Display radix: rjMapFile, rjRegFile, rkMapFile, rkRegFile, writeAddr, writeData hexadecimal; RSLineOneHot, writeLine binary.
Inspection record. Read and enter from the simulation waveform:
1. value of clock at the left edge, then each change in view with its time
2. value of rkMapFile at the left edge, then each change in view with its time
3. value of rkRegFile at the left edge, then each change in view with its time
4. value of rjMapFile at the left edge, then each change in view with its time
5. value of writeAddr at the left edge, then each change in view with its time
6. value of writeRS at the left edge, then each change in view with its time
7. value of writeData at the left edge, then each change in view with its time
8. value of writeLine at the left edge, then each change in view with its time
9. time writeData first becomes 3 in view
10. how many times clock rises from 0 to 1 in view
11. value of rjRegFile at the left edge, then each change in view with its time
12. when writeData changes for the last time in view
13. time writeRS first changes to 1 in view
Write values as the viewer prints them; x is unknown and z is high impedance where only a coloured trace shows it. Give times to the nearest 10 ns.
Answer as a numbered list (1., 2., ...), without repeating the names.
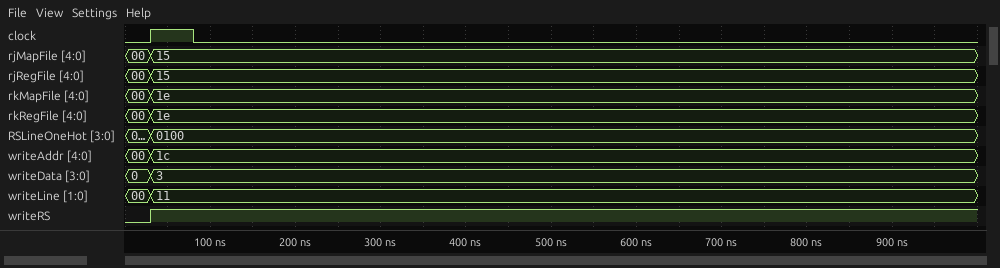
1. 0, 1 at 30 ns, 0 at 80 ns
2. 00, 1e at 30 ns
3. 00, 1e at 30 ns
4. 00, 15 at 30 ns
5. 00, 1c at 30 ns
6. 0, 1 at 30 ns
7. 0, 3 at 30 ns
8. 00, 11 at 30 ns
9. 30 ns
10. 1
11. 00, 15 at 30 ns
12. 30 ns
13. 30 ns
